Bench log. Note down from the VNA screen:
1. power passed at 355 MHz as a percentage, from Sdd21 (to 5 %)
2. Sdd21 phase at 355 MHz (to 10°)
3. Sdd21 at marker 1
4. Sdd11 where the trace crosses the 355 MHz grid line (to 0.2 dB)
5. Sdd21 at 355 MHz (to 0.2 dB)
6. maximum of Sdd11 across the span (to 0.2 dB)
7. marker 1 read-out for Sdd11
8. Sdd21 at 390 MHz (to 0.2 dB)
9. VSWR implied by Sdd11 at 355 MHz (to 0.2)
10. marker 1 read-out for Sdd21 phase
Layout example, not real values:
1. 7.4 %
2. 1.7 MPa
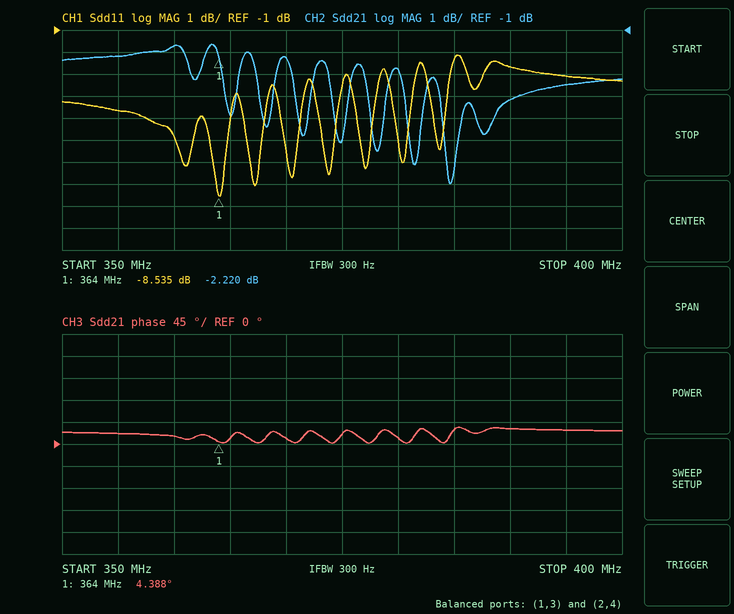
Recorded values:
1. 60 %
2. 20°
3. -2.220 dB
4. -4.6 dB
5. -2.2 dB
6. -2.2 dB
7. -8.535 dB
8. -4.2 dB
9. 3.8
10. 4.388°
